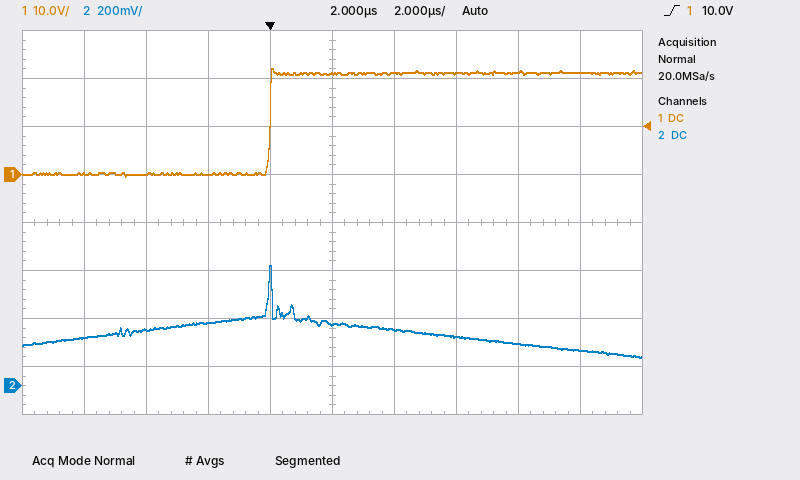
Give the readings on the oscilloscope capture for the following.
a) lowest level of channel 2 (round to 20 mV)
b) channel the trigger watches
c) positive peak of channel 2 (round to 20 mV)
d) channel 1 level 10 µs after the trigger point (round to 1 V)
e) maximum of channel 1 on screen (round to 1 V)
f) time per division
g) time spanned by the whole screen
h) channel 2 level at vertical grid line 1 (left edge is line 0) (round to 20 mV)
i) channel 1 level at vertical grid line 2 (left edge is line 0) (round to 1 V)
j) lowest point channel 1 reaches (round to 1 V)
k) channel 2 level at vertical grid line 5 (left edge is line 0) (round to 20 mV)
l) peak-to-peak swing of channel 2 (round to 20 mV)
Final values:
120 mV
channel 1
500 mV
21 V
22 V
2 µs
20 µs
200 mV
0 V
0 V
260 mV
380 mV
